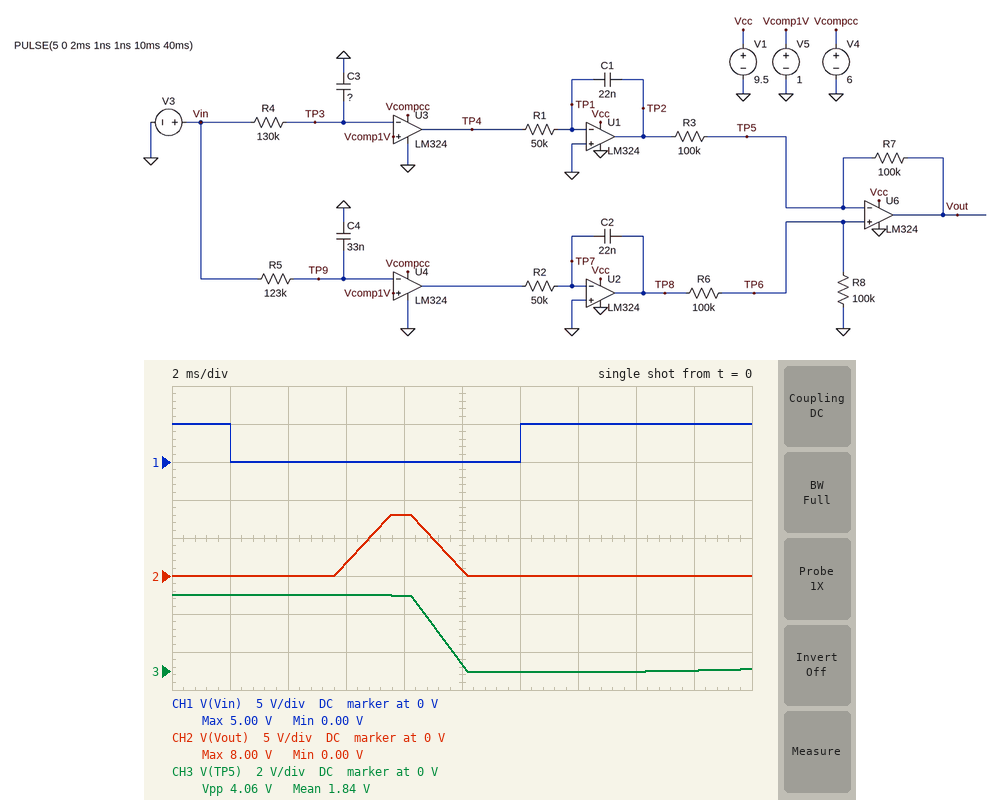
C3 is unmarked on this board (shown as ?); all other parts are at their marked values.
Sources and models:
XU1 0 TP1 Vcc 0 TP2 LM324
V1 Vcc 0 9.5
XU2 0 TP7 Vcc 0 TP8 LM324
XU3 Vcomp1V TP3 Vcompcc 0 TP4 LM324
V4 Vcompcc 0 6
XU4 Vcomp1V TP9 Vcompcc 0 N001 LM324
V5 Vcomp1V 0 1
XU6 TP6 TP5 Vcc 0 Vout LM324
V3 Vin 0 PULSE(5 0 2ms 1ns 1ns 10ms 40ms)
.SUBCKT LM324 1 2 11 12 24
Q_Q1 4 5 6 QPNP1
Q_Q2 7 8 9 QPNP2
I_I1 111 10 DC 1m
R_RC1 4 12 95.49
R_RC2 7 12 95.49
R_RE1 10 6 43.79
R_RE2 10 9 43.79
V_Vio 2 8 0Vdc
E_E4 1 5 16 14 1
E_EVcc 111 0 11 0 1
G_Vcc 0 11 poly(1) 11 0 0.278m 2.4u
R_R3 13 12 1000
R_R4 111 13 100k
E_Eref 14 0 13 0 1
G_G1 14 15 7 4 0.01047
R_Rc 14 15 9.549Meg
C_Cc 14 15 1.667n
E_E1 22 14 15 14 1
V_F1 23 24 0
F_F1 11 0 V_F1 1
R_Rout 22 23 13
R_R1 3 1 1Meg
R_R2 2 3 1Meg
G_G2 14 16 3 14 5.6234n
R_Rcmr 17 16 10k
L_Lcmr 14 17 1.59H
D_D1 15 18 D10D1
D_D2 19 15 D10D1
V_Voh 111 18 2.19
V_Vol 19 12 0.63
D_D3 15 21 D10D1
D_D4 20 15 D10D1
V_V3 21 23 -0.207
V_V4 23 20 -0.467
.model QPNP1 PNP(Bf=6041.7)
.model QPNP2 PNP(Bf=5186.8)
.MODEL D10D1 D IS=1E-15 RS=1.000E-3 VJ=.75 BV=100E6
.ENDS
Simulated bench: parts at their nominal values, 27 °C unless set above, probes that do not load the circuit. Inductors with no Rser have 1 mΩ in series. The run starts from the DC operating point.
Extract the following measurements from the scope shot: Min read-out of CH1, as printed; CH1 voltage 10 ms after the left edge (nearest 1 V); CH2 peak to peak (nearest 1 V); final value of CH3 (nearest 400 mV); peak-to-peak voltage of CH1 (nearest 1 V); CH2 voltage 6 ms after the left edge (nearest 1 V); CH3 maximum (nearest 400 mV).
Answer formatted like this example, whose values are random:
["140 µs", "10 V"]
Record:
["0.00 V", "0 V", "8 V", "0 V", "5 V", "2 V", "4.0 V"]
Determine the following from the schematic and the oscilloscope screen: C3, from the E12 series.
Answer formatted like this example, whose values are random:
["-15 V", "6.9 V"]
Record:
["18 nF"]
